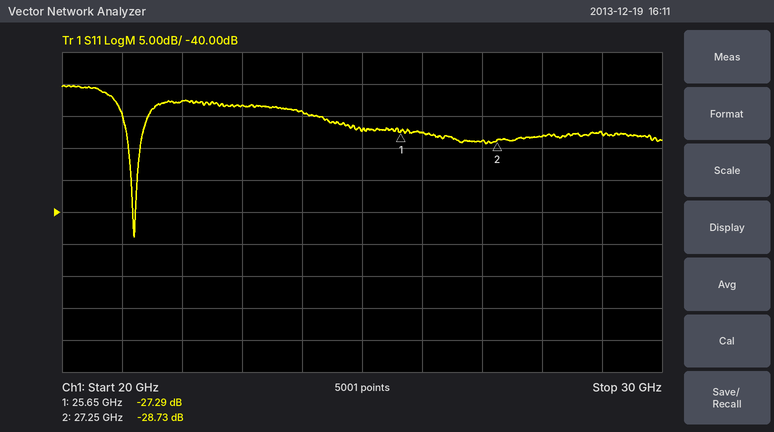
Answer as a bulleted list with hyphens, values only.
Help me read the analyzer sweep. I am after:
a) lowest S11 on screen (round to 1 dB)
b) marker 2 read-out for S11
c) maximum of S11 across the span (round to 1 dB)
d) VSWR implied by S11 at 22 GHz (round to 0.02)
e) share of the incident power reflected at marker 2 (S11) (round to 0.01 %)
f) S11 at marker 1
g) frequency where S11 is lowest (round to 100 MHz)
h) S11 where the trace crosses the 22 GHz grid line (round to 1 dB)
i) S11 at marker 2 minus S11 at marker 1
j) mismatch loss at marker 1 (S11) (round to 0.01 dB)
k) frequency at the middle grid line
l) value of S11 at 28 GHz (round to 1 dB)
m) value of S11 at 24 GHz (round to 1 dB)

- -44 dB
- -28.73 dB
- -20 dB
- 1.16
- 0.13 %
- -27.29 dB
- 21.2 GHz
- -23 dB
- -1.44 dB
- 0.01 dB
- 25 GHz
- -28 dB
- -24 dB
